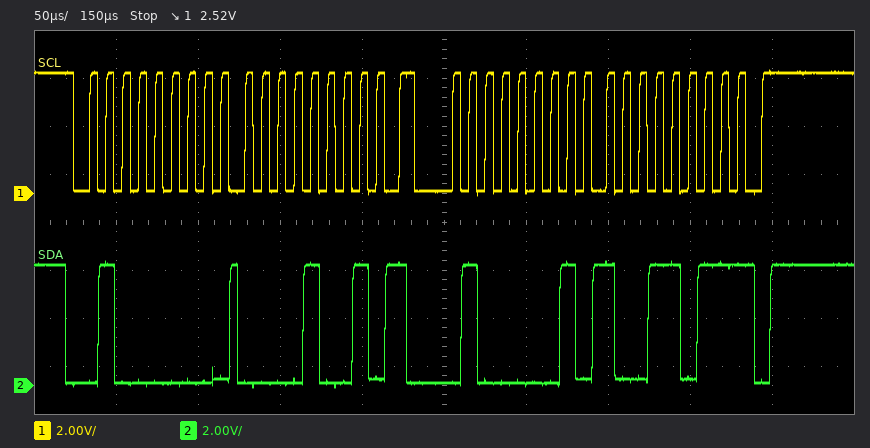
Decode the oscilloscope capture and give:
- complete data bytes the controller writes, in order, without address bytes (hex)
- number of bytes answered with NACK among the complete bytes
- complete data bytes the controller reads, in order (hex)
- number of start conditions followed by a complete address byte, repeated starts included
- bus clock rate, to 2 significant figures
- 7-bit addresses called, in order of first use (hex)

09
1
9B
2
100 kHz
0x20
